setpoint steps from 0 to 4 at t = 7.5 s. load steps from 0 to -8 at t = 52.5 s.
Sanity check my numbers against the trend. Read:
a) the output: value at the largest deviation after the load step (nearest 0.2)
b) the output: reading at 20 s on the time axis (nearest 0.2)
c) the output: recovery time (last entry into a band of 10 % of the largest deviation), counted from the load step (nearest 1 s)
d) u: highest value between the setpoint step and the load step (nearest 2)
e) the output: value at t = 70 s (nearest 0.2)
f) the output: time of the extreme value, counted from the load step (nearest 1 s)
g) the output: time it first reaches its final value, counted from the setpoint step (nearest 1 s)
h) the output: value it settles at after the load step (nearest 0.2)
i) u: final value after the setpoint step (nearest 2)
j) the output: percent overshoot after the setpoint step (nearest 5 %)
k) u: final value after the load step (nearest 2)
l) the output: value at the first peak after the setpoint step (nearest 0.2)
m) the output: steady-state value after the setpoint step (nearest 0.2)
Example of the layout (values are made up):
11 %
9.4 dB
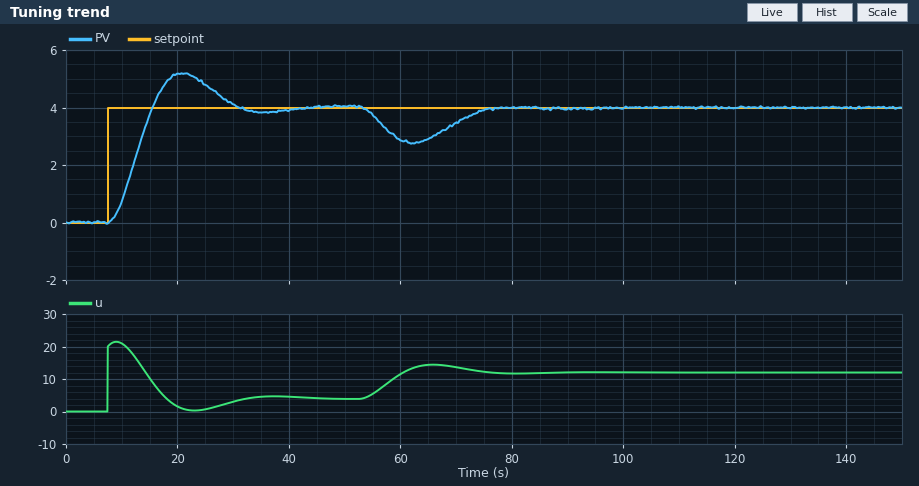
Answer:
2.8
5.2
22 s
22
3.4
10 s
8 s
4.0
4
30 %
12
5.2
4.0
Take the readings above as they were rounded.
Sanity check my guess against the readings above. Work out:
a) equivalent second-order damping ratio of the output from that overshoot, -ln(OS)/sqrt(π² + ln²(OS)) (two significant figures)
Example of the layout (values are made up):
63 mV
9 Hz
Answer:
0.36
